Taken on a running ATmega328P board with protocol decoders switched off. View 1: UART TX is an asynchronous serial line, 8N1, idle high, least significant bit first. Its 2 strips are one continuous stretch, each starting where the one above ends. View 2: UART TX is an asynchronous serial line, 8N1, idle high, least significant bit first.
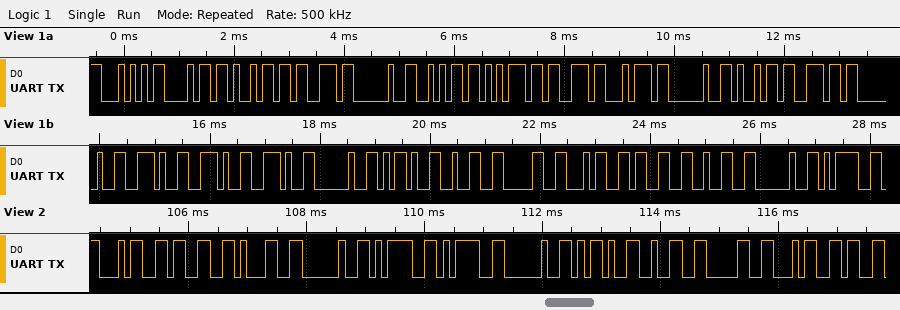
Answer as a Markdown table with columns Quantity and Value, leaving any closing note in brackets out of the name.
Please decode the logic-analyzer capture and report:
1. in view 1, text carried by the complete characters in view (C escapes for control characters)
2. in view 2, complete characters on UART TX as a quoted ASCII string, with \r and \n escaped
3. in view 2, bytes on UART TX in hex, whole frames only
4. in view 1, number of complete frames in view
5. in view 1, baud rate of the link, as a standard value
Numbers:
| Quantity | Value |
|---|---|
| in view 1, text carried by the complete characters in view | "This just in ... -20432 =" |
| in view 2, complete characters on UART TX as a quoted ASCII string, with \r and \n escaped | "431 == -204" |
| in view 2, bytes on UART TX in hex, whole frames only | 34 33 31 20 3D 3D 20 2D 32 30 34 |
| in view 1, number of complete frames in view | 25 |
| in view 1, baud rate of the link, as a standard value | 9600 baud |
